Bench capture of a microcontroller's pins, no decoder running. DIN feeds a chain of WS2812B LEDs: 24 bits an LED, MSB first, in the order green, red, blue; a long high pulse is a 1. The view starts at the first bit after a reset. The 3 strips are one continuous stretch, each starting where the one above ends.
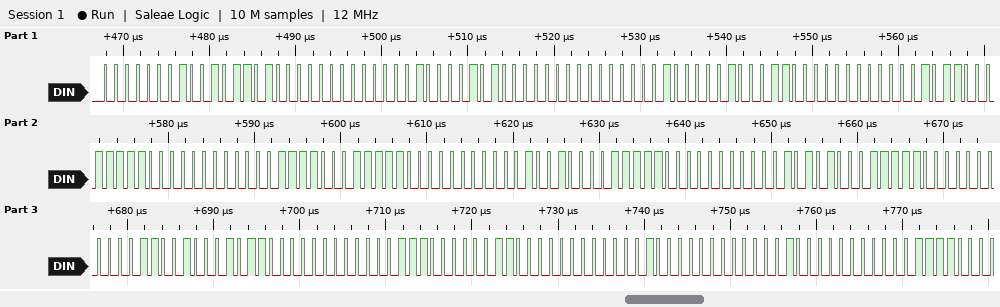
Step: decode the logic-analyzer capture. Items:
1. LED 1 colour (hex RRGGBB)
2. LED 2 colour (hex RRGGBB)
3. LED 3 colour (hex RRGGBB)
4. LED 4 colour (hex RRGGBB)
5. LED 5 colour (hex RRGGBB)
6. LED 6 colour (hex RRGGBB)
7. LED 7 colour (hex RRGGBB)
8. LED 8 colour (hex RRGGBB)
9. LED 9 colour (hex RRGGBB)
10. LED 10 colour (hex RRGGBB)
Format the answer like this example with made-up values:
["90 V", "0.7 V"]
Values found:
["#2D0100", "#280400", "#230800", "#1F0B00", "#1F0F00", "#1F1200", "#1F1500", "#161900", "#0C1C00", "#012000"]
